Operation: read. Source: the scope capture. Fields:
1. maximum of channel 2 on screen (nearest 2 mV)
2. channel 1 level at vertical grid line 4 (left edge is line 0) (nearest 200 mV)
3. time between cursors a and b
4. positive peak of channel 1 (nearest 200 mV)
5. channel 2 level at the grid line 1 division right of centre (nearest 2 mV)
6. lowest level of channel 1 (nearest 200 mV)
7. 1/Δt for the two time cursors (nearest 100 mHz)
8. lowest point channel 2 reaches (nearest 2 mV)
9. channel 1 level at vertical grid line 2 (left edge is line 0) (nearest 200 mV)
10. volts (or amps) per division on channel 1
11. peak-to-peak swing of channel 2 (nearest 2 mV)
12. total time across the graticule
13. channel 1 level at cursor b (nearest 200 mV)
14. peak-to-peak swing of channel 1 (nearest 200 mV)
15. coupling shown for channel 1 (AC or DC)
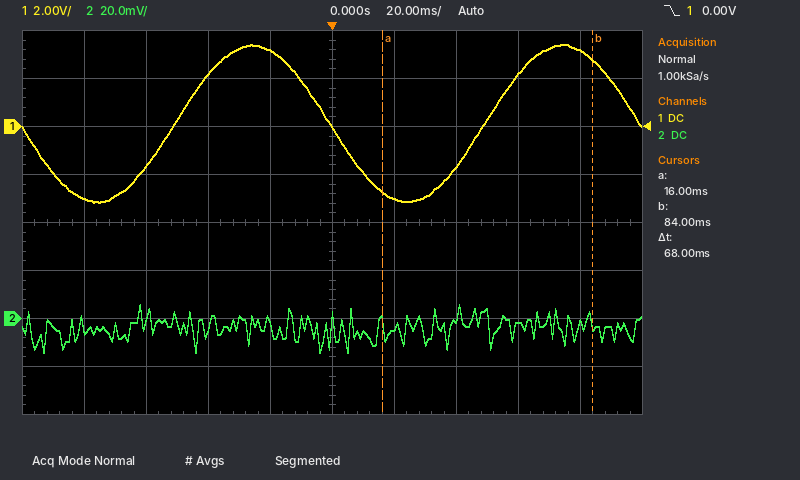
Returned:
6 mV
3.2 V
68 ms
3.4 V
-4 mV
-3.2 V
14.7 Hz
-14 mV
-1.6 V
2 V
20 mV
200 ms
2.8 V
6.6 V
DC
